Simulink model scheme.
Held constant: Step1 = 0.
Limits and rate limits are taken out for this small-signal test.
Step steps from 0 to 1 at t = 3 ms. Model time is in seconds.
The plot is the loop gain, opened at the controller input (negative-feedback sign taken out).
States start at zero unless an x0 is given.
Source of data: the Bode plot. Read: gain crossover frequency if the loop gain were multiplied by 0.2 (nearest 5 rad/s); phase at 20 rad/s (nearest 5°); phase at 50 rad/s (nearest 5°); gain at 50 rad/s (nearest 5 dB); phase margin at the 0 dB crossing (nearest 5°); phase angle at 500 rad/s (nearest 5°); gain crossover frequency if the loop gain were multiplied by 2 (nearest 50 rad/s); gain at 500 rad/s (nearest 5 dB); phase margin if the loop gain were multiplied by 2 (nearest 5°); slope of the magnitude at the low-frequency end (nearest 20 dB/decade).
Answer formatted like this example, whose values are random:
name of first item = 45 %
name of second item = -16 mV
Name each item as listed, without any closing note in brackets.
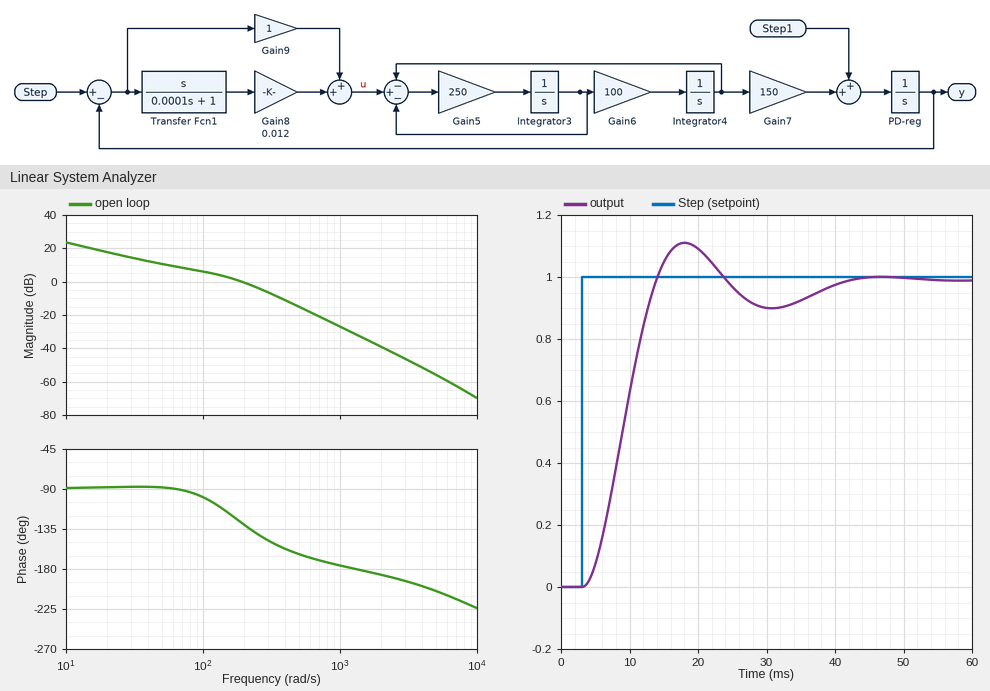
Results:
gain crossover frequency if the loop gain were multiplied by 0.2 = 30 rad/s
phase at 20 rad/s = -90°
phase at 50 rad/s = -90°
gain at 50 rad/s = 10 dB
phase margin at the 0 dB crossing = 50°
phase angle at 500 rad/s = -165°
gain crossover frequency if the loop gain were multiplied by 2 = 300 rad/s
gain at 500 rad/s = -15 dB
phase margin if the loop gain were multiplied by 2 = 35°
slope of the magnitude at the low-frequency end = -20 dB/decade
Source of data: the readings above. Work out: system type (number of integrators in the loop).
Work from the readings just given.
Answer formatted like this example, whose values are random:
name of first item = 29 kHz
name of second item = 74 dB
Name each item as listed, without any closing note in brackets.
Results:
system type = 1
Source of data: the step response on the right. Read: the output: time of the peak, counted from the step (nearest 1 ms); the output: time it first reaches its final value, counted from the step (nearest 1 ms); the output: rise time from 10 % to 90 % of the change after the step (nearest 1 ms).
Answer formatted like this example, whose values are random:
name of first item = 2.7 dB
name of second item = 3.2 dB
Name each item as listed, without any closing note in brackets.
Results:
the output: time of the peak, counted from the step = 15 ms
the output: time it first reaches its final value, counted from the step = 11 ms
the output: rise time from 10 % to 90 % of the change after the step = 7 ms
